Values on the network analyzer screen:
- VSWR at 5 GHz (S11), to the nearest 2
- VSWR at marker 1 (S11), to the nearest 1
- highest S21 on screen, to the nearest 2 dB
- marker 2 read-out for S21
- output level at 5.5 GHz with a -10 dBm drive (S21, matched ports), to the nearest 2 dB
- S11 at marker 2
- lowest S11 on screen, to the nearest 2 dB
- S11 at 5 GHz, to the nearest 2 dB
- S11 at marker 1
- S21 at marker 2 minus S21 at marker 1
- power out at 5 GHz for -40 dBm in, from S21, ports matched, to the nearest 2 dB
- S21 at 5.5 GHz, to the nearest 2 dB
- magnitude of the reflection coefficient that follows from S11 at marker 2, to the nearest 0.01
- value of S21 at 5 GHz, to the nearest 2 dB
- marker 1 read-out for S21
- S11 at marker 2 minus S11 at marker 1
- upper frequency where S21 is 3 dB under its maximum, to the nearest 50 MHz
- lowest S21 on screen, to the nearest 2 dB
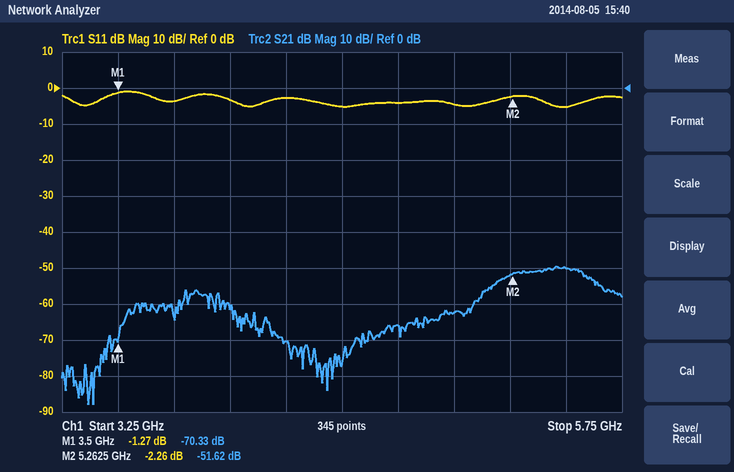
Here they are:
4
14
-50 dB
-51.62 dB
-60 dBm
-2.26 dB
-6 dB
-4 dB
-1.27 dB
18.71 dB
-102 dBm
-50 dB
0.77
-62 dB
-70.33 dB
-0.99 dB
5.60 GHz
-88 dB
